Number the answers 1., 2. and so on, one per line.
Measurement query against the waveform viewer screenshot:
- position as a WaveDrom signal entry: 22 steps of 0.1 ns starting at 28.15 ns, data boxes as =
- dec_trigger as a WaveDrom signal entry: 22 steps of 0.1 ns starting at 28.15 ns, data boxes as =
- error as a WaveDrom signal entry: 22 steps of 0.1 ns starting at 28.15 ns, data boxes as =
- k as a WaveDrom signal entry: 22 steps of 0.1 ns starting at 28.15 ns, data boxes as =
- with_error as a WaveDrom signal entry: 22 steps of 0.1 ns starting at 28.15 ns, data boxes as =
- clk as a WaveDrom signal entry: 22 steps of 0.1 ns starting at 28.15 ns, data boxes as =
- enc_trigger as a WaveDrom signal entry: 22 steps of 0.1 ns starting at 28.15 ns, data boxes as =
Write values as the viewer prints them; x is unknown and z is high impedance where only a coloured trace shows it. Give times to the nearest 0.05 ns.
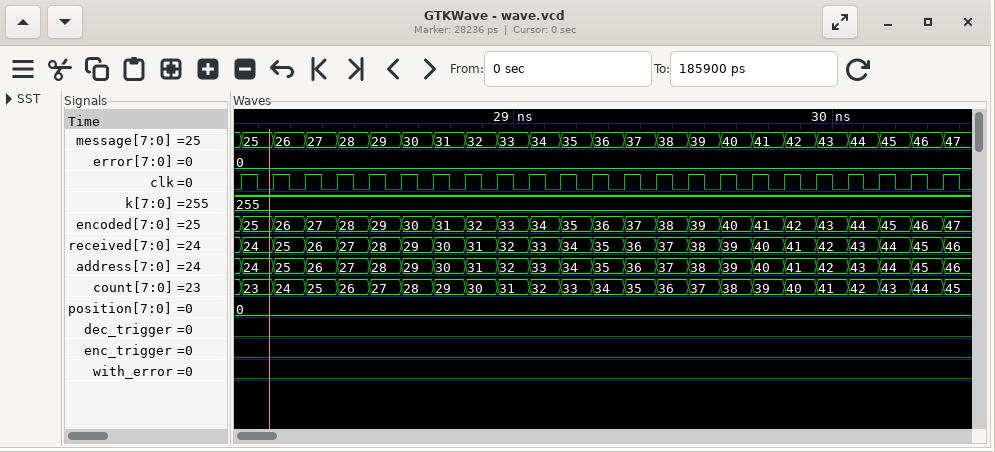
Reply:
1. {name: 'position', wave: '=.....................', data: '0'}
2. {name: 'dec_trigger', wave: '0.....................'}
3. {name: 'error', wave: '=.....................', data: '0'}
4. {name: 'k', wave: '=.....................', data: '255'}
5. {name: 'with_error', wave: '0.....................'}
6. {name: 'clk', wave: 'p.....................'}
7. {name: 'enc_trigger', wave: '0.....................'}
